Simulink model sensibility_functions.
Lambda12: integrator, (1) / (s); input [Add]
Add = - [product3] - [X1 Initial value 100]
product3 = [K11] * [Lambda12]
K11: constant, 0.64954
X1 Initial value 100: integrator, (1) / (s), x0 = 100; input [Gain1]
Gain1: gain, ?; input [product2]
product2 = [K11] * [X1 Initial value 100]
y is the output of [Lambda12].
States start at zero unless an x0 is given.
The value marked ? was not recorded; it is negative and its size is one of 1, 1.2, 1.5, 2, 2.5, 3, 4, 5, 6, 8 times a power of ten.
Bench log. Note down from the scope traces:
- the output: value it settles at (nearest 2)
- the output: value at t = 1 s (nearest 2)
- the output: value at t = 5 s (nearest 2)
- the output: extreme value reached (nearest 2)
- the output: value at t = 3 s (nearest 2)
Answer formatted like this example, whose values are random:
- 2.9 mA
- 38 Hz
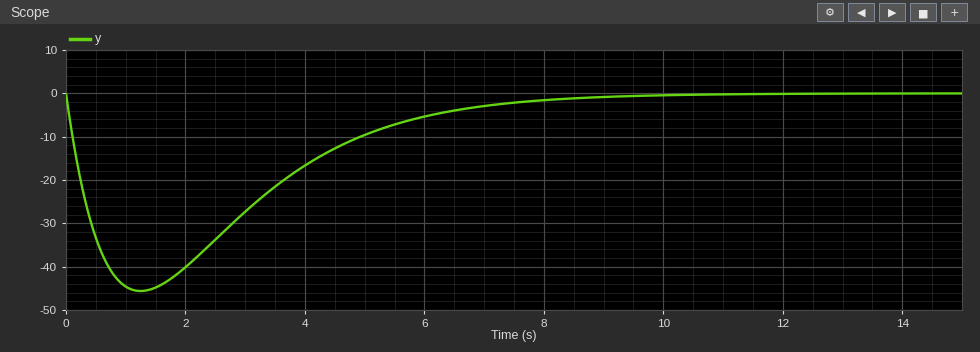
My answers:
- 0
- -44
- -10
- -46
- -28
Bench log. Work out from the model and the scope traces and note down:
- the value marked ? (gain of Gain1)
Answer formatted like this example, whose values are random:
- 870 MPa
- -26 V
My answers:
- -1.5
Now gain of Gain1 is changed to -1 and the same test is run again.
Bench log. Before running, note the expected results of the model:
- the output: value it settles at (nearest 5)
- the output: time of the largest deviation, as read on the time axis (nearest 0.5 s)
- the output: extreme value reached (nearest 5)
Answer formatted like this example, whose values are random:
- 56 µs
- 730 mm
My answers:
- 0
- 1.5 s
- -55
